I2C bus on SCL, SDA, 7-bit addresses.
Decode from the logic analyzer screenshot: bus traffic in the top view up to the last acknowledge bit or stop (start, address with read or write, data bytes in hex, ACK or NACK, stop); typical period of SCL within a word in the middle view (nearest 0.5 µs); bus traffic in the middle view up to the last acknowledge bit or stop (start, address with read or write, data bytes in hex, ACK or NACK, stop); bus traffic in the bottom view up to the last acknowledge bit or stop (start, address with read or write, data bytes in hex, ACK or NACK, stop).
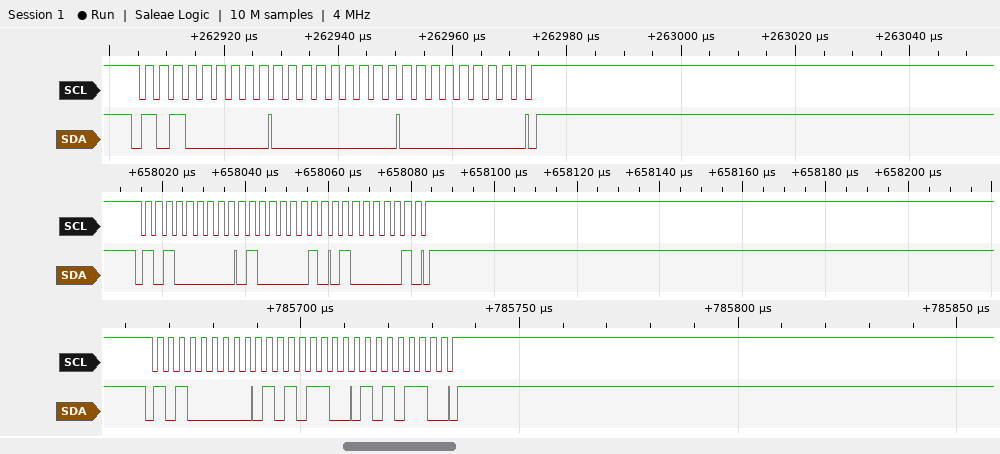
start, address 50 write ACK, 00 ACK, 00 ACK, stop
2.5 µs
start, address 50 write ACK, 41 ACK, 41 ACK, stop
start, address 50 write ACK, 56 ACK, 56 ACK, stop
